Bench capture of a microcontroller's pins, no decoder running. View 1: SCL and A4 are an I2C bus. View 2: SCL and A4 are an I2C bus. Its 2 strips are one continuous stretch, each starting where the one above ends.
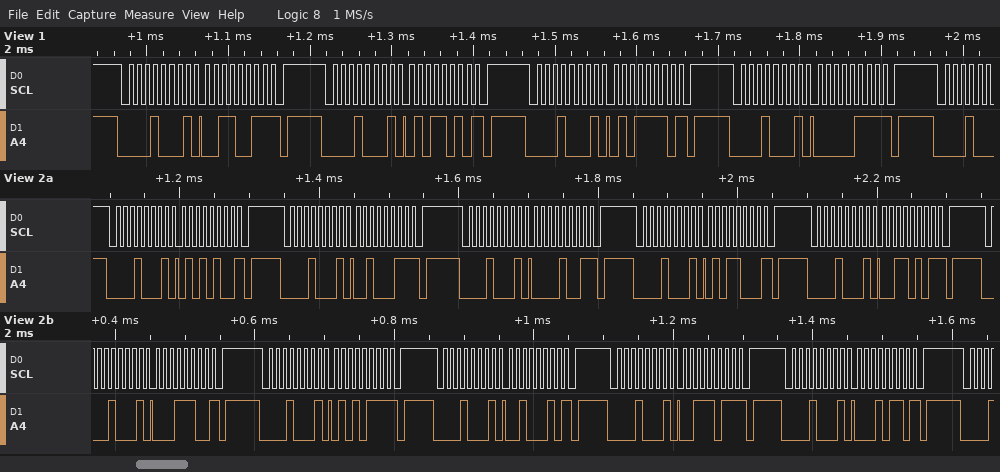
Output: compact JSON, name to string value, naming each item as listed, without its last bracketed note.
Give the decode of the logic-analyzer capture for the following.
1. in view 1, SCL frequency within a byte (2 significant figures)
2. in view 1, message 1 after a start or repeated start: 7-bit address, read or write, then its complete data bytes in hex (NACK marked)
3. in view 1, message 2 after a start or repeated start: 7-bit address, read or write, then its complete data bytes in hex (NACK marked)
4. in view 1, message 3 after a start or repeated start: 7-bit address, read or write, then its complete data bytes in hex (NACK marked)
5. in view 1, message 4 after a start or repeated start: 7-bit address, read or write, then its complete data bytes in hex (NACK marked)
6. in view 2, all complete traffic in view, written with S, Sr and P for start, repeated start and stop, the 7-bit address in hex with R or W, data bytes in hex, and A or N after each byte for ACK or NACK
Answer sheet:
{"in view 1, SCL frequency within a byte": "100 kHz", "in view 1, message 1 after a start or repeated start: 7-bit address, read or write, then its complete data bytes in hex": "0x08 read: 33 NACK", "in view 1, message 2 after a start or repeated start: 7-bit address, read or write, then its complete data bytes in hex": "0x08 read: 5A NACK", "in view 1, message 3 after a start or repeated start: 7-bit address, read or write, then its complete data bytes in hex": "0x08 read: 5E NACK", "in view 1, message 4 after a start or repeated start: 7-bit address, read or write, then its complete data bytes in hex": "0x08 read: 07 NACK", "in view 2, all complete traffic in view, written with S, Sr and P for start, repeated start and stop, the 7-bit address in hex with R or W, data bytes in hex, and A or N after each byte for ACK or NACK": "S 08R A 54 N P S 08R A 23 N P S 08R A 09 N P S 08R A 58 N P S 08R A 35 N P S 08R A 1C N P S 08R A 57 N P S 08R A 22 N P S 08R A 3B N P S 08R A 16 N P"}
